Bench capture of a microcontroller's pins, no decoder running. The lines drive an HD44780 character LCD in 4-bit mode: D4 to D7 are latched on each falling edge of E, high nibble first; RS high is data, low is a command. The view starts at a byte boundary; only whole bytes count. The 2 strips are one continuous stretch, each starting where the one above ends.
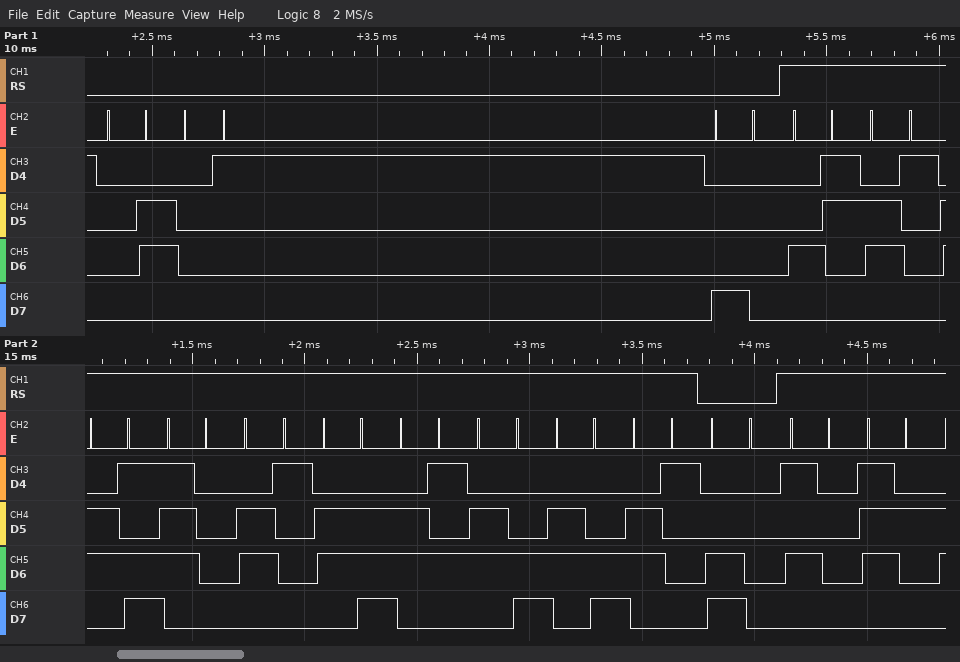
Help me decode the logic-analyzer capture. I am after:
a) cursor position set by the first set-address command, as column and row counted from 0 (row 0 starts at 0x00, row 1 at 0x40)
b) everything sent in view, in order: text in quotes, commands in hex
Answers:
column 0, row 0
0x06 0x01 0x80 "Campanella" 0xC0 "Pr"
